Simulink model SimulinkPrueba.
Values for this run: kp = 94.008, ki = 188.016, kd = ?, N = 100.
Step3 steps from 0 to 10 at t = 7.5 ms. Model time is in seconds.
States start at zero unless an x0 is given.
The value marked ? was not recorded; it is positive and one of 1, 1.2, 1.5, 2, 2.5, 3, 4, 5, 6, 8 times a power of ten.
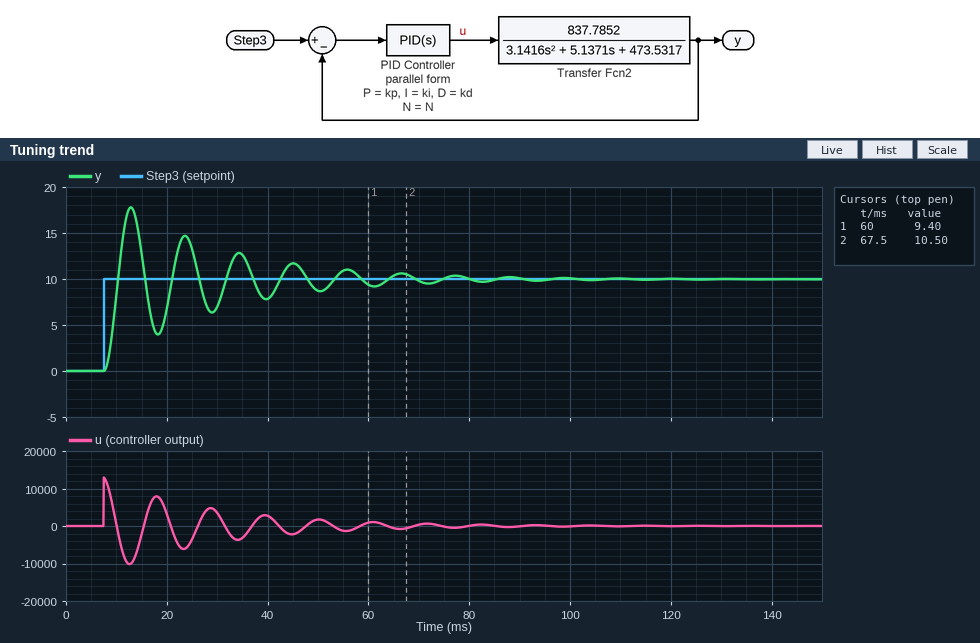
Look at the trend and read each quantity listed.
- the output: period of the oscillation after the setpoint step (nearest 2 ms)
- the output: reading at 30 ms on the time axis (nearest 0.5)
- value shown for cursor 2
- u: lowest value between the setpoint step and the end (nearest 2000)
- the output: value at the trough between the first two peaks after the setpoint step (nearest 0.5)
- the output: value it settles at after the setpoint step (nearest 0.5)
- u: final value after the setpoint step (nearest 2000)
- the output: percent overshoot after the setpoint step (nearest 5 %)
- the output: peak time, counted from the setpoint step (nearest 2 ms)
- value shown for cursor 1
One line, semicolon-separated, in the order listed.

10 ms; 7.0; 10.50; -10000; 4.0; 10.0; 0; 80 %; 6 ms; 9.40
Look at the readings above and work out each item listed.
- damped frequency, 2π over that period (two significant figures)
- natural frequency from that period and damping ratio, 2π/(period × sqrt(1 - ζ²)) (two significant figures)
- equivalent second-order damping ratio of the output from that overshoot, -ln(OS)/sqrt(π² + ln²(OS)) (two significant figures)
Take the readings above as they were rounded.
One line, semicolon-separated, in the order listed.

0.63 rad/ms; 0.63 rad/ms; 0.071
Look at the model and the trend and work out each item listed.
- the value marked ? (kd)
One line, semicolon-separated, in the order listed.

12
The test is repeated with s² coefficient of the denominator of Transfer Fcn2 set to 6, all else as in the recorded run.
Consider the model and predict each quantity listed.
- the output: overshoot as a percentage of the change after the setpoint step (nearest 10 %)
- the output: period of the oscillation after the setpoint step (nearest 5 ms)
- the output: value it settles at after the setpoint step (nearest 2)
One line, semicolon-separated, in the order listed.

70 %; 15 ms; 10
